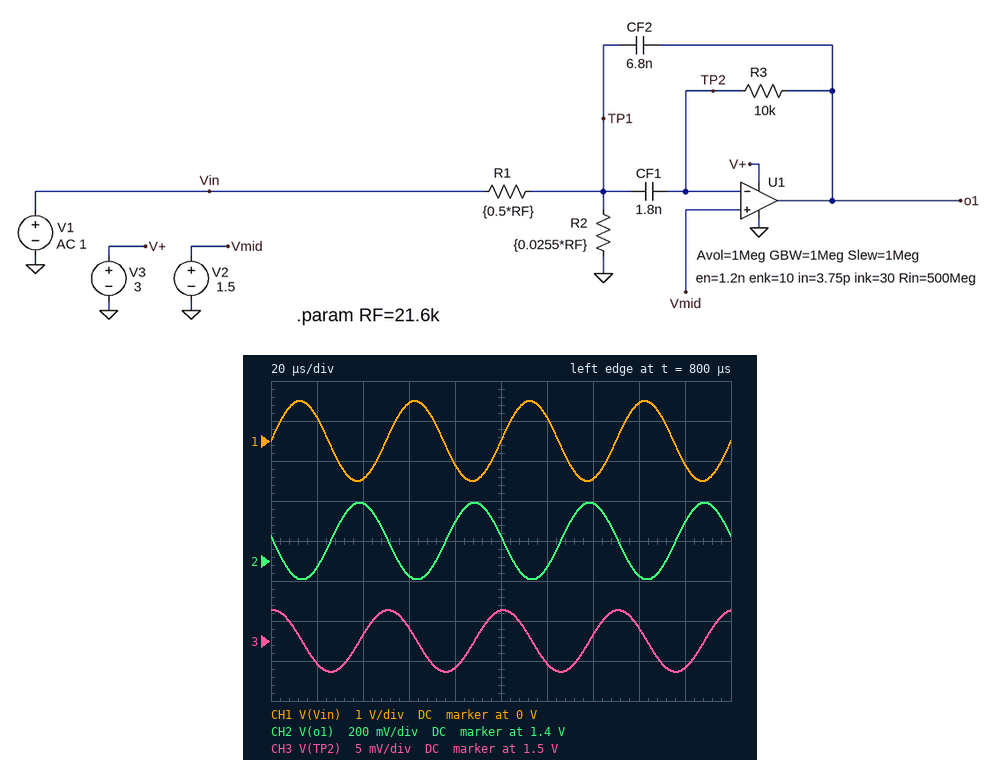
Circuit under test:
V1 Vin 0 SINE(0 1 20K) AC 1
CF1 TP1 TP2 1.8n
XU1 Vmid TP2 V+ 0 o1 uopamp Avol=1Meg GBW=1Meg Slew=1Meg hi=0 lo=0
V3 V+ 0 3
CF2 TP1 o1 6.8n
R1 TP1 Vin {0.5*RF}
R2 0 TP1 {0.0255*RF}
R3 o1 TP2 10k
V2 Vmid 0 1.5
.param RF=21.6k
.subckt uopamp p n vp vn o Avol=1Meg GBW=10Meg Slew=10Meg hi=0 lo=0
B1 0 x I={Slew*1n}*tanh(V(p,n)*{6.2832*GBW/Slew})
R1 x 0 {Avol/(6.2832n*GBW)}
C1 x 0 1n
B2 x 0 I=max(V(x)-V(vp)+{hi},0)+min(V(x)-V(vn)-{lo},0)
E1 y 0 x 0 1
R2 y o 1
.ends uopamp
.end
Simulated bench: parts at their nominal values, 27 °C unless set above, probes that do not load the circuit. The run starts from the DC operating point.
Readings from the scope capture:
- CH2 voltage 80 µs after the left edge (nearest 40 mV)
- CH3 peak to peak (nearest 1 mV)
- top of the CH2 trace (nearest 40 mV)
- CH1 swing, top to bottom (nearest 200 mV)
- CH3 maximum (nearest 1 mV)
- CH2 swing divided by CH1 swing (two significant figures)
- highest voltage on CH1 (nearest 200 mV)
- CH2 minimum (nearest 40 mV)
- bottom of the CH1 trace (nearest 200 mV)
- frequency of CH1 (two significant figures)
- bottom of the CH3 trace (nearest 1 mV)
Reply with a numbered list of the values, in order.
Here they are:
1. 1.60 V
2. 8 mV
3. 1.68 V
4. 2.0 V
5. 1.504 V
6. 0.19
7. 1.0 V
8. 1.32 V
9. -1.0 V
10. 20 kHz
11. 1.496 V
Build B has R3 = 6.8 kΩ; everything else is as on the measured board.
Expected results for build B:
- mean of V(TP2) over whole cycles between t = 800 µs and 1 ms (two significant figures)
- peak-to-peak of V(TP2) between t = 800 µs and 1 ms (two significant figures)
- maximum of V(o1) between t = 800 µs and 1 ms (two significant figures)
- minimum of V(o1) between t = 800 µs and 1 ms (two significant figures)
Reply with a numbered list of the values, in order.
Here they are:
1. 1.5 V
2. 4.7 mV
3. 1.6 V
4. 1.4 V
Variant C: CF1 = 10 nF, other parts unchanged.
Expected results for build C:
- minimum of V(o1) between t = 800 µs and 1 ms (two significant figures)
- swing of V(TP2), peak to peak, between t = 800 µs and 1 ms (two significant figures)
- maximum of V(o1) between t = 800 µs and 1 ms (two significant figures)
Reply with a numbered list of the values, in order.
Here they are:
1. 1.4 V
2. 4.9 mV
3. 1.6 V
